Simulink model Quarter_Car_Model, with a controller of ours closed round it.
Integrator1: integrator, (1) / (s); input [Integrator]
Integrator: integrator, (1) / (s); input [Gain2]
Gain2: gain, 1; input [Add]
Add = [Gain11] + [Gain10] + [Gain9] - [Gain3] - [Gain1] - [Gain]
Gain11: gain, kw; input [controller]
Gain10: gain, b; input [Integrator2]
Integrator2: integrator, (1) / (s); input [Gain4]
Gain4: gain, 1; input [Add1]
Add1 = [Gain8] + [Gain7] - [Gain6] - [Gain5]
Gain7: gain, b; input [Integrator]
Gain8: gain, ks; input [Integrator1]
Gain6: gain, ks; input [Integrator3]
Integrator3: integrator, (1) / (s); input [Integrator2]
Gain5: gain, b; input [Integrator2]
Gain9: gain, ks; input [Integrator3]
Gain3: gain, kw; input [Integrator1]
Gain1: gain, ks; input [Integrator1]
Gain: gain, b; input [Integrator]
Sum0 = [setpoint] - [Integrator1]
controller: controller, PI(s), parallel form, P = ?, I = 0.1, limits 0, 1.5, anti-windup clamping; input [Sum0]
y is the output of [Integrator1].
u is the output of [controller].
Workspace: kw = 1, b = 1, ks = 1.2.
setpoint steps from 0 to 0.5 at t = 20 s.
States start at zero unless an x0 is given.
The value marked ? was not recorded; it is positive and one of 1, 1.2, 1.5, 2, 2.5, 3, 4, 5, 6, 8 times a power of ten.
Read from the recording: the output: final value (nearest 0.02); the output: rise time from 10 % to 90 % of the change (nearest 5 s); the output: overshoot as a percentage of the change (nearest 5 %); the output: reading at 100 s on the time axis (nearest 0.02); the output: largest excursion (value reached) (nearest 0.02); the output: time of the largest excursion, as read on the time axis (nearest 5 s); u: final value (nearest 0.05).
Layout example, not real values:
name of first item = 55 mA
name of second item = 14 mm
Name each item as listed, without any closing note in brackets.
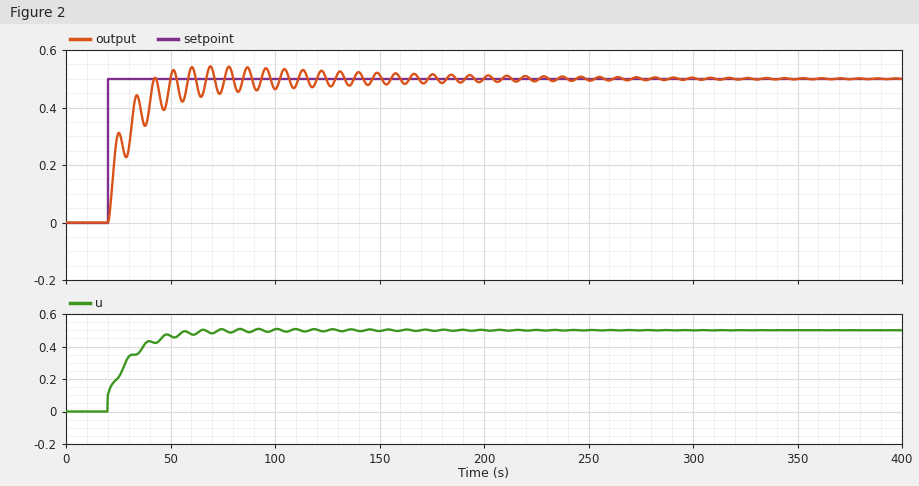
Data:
the output: final value = 0.50
the output: rise time from 10 % to 90 % of the change = 20 s
the output: overshoot as a percentage of the change = 10 %
the output: reading at 100 s on the time axis = 0.46
the output: largest excursion (value reached) = 0.54
the output: time of the largest excursion, as read on the time axis = 70 s
u: final value = 0.50
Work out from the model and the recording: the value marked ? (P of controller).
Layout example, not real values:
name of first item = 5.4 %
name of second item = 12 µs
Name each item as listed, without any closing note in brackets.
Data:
the value marked ? = 0.2
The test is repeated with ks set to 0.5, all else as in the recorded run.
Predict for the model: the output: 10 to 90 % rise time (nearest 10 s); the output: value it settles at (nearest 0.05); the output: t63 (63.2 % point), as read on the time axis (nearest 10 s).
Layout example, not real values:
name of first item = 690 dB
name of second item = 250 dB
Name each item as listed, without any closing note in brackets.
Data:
the output: 10 to 90 % rise time = 30 s
the output: value it settles at = 0.50
the output: t63 (63.2 % point), as read on the time axis = 30 s
